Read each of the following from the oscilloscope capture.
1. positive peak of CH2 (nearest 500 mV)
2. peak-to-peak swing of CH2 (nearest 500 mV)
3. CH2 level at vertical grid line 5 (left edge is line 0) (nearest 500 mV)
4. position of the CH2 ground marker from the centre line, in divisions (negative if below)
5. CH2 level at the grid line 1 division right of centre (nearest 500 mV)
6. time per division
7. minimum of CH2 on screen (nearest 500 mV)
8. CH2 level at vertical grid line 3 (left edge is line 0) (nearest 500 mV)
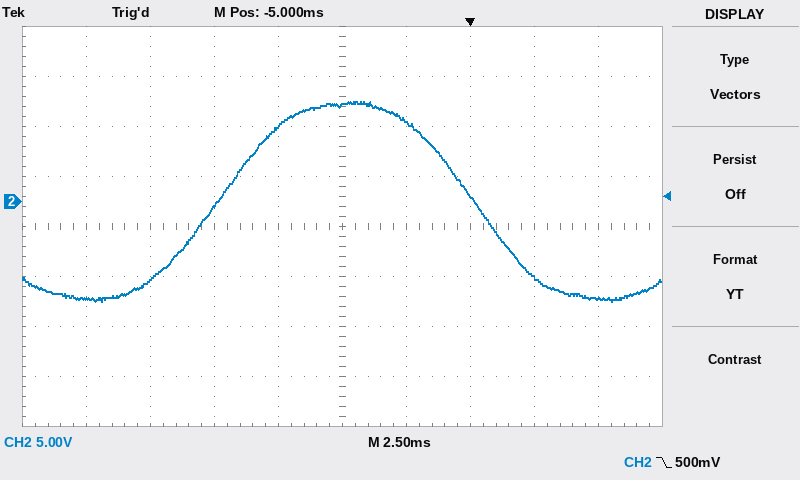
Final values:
10.0 V
20.0 V
9.5 V
+0.5 div
8.0 V
2.5 ms
-10.0 V
-500 mV
